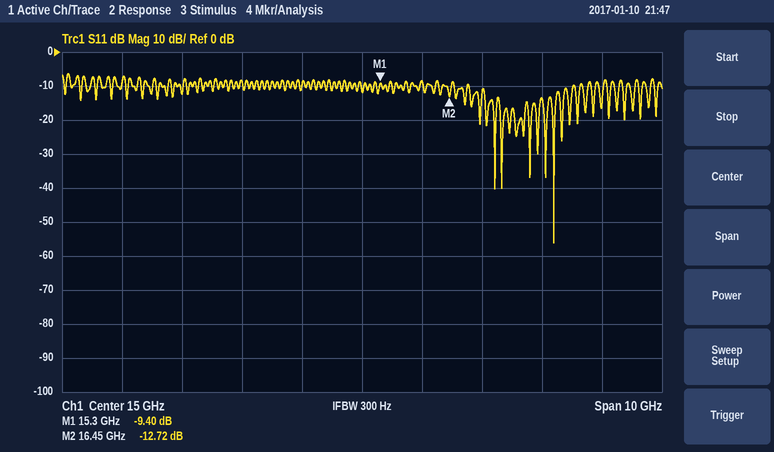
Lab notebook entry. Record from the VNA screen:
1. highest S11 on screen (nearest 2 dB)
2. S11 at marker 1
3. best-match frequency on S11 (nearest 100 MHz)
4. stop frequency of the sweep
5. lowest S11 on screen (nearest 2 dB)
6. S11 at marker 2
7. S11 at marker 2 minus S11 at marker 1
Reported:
-6 dB
-9.40 dB
18.2 GHz
20 GHz
-56 dB
-12.72 dB
-3.32 dB
